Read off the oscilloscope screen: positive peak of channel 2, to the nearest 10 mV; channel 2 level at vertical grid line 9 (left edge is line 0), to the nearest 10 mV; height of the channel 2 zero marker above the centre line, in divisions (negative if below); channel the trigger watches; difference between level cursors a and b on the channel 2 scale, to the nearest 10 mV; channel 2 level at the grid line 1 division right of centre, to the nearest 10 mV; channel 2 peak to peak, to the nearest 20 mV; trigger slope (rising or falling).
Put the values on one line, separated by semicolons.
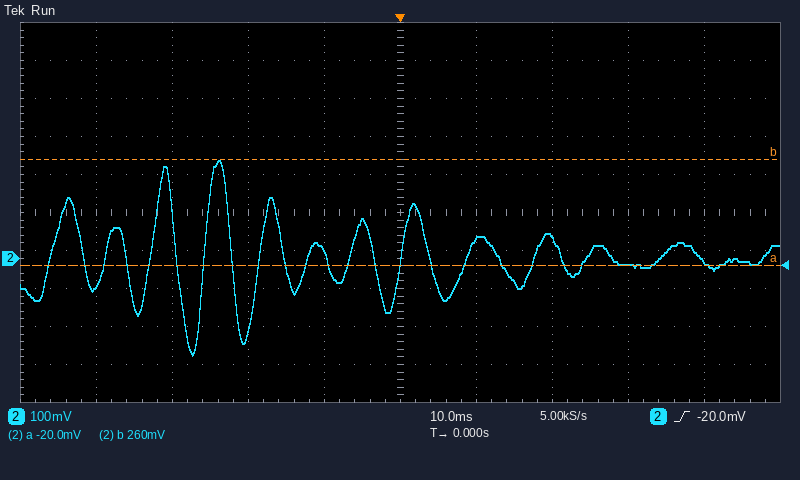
260 mV; -10 mV; -1.2 div; channel 2; 280 mV; 50 mV; 520 mV; rising
